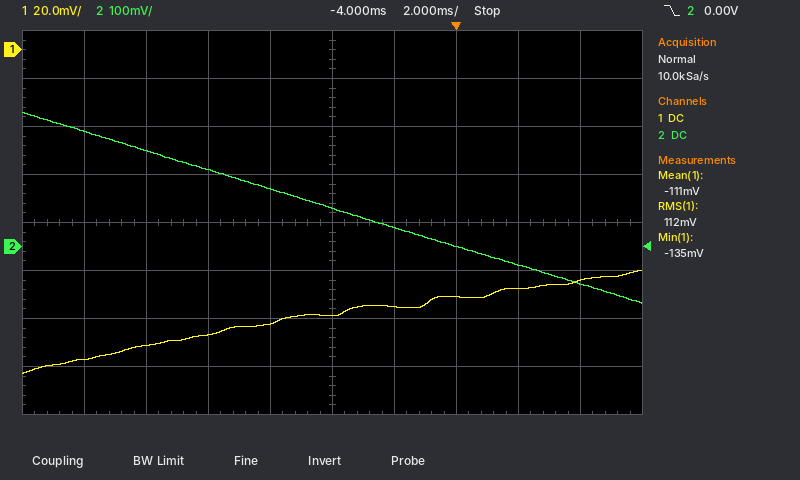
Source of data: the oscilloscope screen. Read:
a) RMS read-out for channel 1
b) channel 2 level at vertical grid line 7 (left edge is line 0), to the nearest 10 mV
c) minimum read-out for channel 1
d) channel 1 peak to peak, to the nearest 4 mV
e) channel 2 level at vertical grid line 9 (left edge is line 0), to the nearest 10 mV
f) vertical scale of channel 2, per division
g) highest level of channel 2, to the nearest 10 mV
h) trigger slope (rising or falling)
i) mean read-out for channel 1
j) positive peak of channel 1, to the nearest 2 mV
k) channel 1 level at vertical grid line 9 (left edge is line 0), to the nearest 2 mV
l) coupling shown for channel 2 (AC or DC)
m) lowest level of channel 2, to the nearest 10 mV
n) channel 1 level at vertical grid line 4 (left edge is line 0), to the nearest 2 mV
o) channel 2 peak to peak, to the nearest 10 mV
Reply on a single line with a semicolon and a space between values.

112 mV; 0 mV; -135 mV; 44 mV; -80 mV; 100 mV; 280 mV; falling; -111 mV; -92 mV; -96 mV; DC; -120 mV; -114 mV; 400 mV
